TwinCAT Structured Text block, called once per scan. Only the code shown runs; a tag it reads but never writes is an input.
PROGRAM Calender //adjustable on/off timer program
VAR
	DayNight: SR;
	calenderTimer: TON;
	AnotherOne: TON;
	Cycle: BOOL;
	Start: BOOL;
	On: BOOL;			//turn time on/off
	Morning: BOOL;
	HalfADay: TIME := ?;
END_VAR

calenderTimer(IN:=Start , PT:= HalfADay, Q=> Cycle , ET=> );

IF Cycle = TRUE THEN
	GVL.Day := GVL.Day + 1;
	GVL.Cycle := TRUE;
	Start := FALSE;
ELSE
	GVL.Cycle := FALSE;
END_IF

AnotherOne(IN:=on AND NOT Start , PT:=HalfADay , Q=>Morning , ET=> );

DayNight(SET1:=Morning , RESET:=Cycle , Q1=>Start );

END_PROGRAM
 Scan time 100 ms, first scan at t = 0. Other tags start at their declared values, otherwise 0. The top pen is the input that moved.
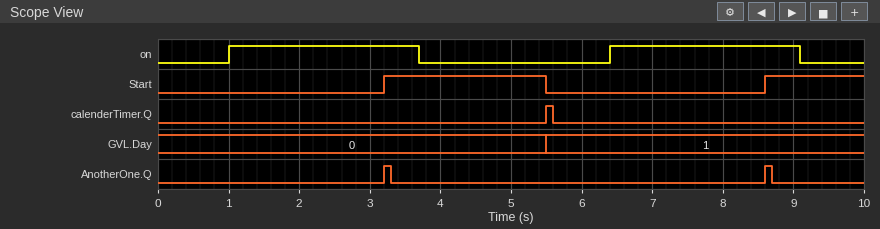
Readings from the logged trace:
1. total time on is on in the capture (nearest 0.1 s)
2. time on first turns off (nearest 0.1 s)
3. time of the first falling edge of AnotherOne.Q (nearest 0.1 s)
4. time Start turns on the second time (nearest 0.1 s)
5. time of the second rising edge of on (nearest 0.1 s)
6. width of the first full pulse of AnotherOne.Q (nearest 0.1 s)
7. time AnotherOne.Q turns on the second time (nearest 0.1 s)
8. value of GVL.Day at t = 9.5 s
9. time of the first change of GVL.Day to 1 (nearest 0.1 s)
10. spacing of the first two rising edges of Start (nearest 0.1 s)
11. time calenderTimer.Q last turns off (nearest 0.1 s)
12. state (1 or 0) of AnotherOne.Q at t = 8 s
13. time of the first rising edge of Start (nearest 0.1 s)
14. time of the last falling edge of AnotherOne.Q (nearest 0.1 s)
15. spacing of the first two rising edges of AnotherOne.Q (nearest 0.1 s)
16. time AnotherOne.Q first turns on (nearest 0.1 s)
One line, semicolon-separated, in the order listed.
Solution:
5.4 s; 3.7 s; 3.3 s; 8.6 s; 6.4 s; 0.1 s; 8.6 s; 1; 5.5 s; 5.4 s; 5.6 s; 0; 3.2 s; 8.7 s; 5.4 s; 3.2 s
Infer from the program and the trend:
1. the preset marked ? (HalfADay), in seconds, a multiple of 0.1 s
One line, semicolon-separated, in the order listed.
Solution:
2.2 s
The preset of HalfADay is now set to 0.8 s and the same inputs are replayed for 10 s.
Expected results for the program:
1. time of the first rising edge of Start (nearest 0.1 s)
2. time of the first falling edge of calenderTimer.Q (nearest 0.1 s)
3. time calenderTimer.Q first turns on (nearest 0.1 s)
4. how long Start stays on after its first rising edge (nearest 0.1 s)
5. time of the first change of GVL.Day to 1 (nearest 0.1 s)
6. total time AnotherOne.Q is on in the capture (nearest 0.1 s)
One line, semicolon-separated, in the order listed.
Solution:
1.8 s; 2.8 s; 2.7 s; 0.9 s; 2.7 s; 0.4 s
